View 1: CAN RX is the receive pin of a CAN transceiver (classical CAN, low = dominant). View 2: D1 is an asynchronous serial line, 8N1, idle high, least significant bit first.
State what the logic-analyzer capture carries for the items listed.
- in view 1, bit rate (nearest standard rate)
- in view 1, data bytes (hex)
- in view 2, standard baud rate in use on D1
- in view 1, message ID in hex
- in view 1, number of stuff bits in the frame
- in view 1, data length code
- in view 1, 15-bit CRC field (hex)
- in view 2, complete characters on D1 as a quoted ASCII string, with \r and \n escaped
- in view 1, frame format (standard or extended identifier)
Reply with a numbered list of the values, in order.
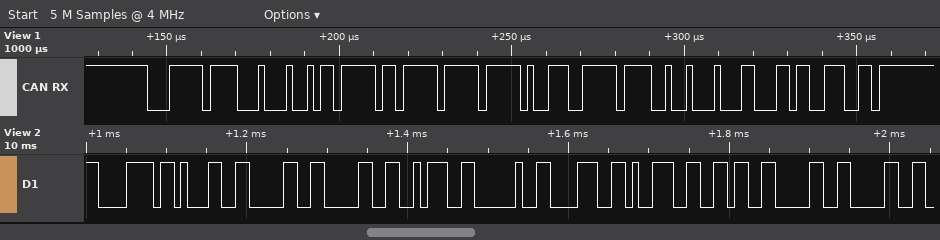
1. 500 kbit/s
2. 96 FE FF FF 39 FF 24 46
3. 115200 baud
4. 0x1FF
5. 6
6. 8
7. 0x1B39
8. "x100: 89600"
9. standard
